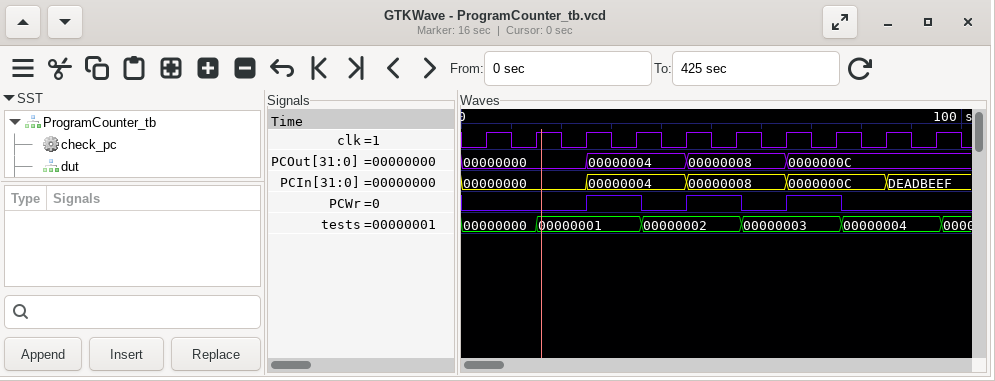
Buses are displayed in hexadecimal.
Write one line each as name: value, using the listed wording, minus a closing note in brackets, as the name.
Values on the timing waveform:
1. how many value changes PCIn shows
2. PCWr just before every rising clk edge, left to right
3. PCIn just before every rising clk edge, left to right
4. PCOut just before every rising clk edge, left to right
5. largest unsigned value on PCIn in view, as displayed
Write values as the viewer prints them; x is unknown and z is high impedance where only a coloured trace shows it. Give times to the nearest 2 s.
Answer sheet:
how many value changes PCIn shows: 4
PCWr just before every rising clk edge, left to right: 0 0 0 1 0 1 0 1 0 0
PCIn just before every rising clk edge, left to right: 00000000, 00000000, 00000000, 00000004, 00000004, 00000008, 00000008, 0000000C, 0000000C, DEADBEEF
PCOut just before every rising clk edge, left to right: 00000000, 00000000, 00000000, 00000004, 00000004, 00000008, 00000008, 0000000C, 0000000C, 0000000C
largest unsigned value on PCIn in view, as displayed: DEADBEEF
